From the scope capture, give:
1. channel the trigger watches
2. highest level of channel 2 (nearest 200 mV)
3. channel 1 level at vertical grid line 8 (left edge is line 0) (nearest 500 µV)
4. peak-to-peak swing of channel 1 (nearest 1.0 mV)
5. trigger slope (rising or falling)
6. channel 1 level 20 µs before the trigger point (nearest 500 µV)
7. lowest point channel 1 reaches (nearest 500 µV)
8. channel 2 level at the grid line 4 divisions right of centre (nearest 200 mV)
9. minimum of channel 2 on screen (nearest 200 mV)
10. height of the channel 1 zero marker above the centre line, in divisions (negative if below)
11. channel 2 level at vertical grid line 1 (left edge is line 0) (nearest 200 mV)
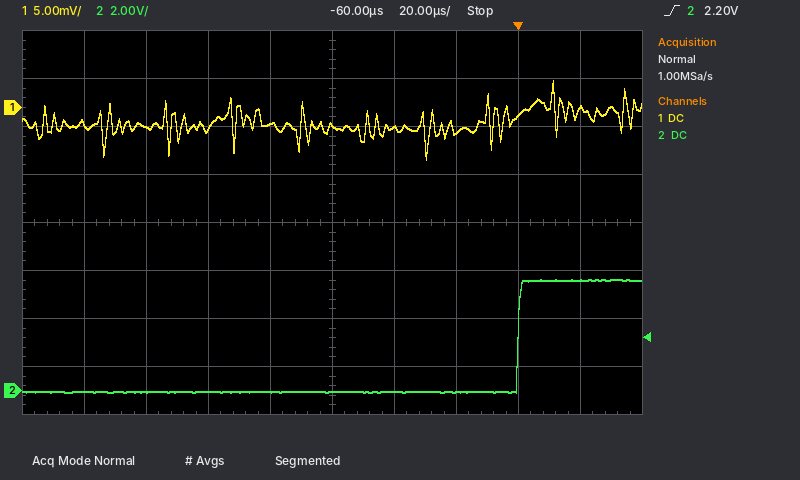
channel 2
4.6 V
-1.0 mV
8.0 mV
rising
-2.5 mV
-5.5 mV
4.6 V
0.0 V
+2.4 div
0.0 V
